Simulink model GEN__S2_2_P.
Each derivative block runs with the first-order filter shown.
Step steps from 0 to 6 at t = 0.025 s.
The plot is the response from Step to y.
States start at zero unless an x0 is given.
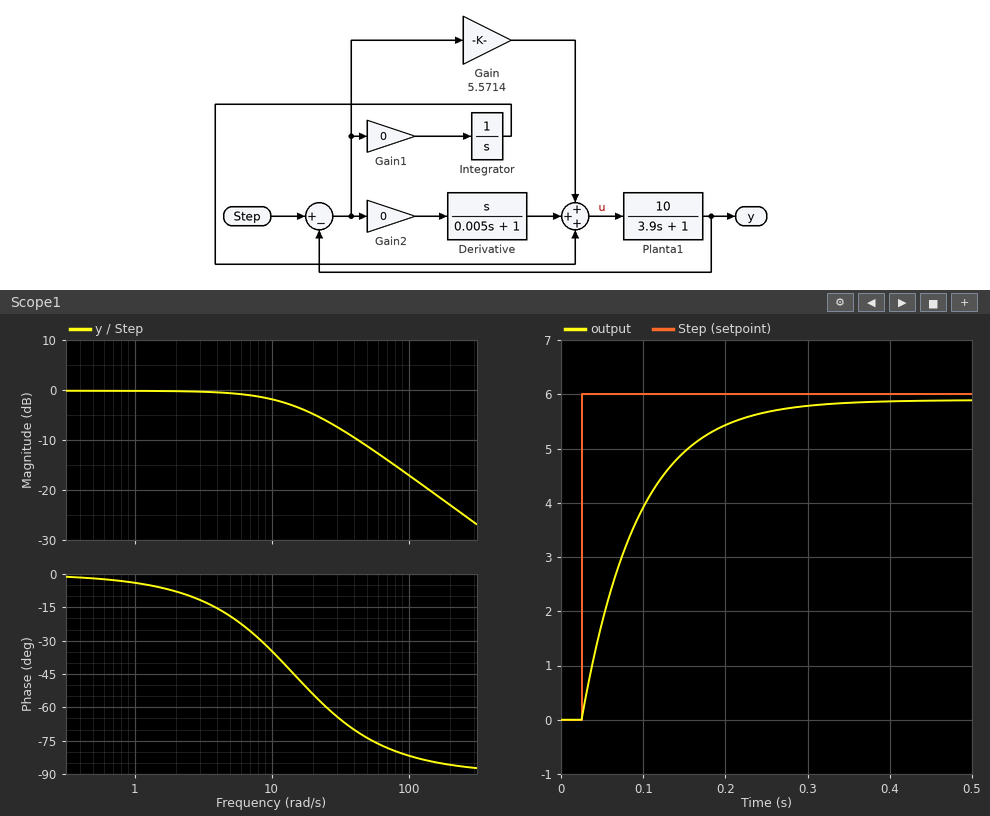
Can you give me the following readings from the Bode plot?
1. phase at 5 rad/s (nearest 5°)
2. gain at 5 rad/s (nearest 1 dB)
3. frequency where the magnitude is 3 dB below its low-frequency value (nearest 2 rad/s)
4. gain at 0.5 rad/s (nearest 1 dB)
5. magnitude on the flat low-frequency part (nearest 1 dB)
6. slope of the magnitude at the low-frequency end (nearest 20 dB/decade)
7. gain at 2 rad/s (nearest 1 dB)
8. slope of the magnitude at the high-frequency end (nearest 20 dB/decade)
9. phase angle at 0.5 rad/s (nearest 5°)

-20°
-1 dB
14 rad/s
0 dB
0 dB
0 dB/decade
0 dB
-20 dB/decade
0°
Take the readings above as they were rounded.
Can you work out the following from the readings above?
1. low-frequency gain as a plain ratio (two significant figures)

1.0
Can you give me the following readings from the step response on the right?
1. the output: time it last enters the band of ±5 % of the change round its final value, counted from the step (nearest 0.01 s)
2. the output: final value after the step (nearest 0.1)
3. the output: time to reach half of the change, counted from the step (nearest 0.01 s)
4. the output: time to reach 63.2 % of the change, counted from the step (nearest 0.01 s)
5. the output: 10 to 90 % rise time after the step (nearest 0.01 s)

0.21 s
5.9
0.05 s
0.07 s
0.15 s
